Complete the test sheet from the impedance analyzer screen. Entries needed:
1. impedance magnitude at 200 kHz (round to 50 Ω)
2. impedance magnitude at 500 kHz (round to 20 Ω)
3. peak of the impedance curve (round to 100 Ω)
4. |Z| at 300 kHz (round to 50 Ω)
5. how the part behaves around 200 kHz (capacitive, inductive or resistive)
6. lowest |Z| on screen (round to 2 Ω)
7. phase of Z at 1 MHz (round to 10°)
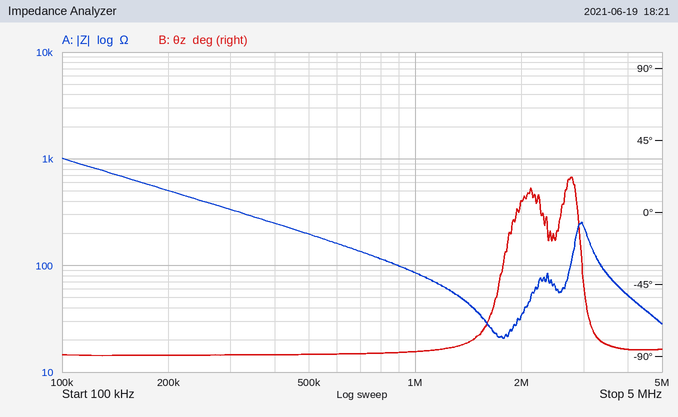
500 Ω
200 Ω
1.0 kΩ
350 Ω
capacitive
20 Ω
-90°
